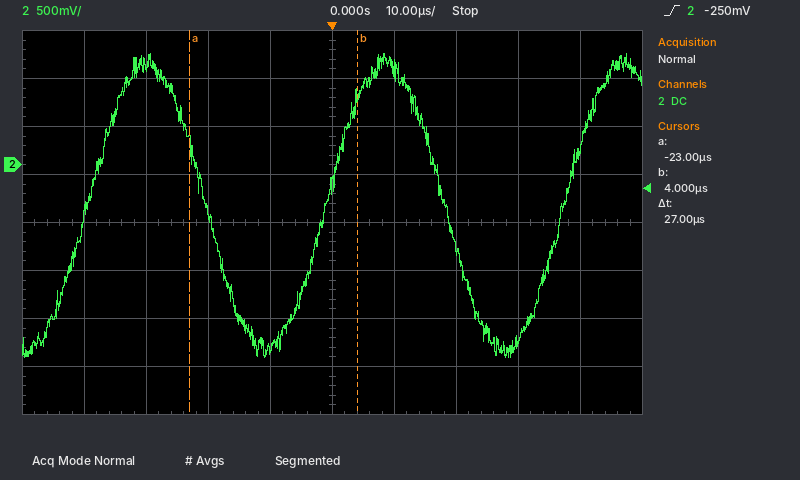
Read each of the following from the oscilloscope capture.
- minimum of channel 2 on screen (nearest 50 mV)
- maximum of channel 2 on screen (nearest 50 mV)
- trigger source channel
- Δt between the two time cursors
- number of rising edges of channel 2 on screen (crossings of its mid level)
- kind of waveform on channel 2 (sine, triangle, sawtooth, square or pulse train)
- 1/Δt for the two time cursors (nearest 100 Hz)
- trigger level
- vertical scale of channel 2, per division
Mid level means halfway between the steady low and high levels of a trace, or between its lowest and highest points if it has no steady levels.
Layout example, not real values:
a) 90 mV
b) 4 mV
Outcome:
a) -2.00 V
b) 1.15 V
c) channel 2
d) 27 µs
e) 3
f) sine
g) 37.0 kHz
h) -250 mV
i) 500 mV
